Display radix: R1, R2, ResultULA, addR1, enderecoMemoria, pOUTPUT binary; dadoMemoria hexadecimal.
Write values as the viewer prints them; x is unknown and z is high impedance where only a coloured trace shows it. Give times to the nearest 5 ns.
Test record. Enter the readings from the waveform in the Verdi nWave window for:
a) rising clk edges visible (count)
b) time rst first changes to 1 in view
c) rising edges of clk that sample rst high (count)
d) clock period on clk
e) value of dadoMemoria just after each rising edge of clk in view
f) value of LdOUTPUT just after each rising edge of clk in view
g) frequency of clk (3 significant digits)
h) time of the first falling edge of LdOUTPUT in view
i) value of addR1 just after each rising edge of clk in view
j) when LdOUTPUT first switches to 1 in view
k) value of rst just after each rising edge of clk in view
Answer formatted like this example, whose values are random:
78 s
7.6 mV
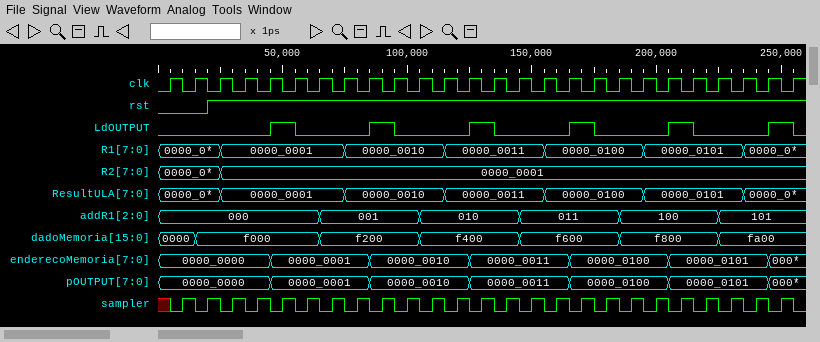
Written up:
26
20 ns
24
10 ns
0000, f000, f000, f000, f000, f000, f200, f200, f200, f200, f400, f400, f400, f400, f600, f600, f600, f600, f800, f800, f800, f800, fa00, fa00, fa00, fa00
0 0 0 0 1 0 0 0 1 0 0 0 1 0 0 0 1 0 0 0 1 0 0 0 1 0
100 MHz
55 ns
000, 000, 000, 000, 000, 000, 001, 001, 001, 001, 010, 010, 010, 010, 011, 011, 011, 011, 100, 100, 100, 100, 101, 101, 101, 101
45 ns
0 0 1 1 1 1 1 1 1 1 1 1 1 1 1 1 1 1 1 1 1 1 1 1 1 1
